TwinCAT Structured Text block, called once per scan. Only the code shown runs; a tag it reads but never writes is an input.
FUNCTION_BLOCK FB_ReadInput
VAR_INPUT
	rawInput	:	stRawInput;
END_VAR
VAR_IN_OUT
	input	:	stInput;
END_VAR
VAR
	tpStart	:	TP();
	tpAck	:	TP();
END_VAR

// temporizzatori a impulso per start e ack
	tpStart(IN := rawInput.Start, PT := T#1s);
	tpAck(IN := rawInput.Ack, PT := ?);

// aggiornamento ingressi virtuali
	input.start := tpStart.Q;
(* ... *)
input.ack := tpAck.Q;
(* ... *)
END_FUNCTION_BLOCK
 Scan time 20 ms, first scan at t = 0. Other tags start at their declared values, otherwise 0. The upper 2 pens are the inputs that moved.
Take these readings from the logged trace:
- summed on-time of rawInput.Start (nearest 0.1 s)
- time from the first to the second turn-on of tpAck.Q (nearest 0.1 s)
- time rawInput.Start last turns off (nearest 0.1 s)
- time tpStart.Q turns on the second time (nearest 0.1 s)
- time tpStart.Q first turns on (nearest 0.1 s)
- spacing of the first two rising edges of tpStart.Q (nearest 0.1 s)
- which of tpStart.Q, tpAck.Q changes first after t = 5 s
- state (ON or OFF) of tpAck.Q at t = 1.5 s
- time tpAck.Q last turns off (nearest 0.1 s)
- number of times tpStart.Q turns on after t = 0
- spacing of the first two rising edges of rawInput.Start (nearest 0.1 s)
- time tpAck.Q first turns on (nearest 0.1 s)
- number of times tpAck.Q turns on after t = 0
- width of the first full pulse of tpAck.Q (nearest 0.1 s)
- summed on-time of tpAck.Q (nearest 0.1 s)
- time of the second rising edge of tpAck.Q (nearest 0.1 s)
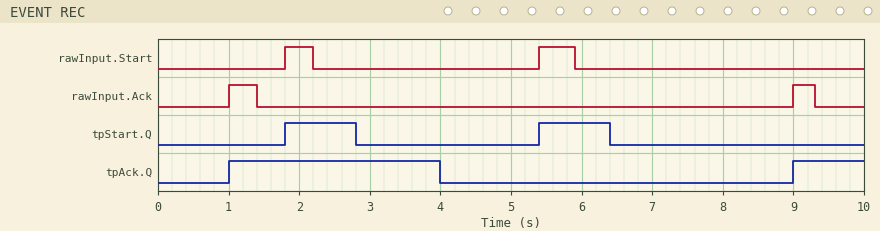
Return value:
0.9 s
8.0 s
5.9 s
5.4 s
1.8 s
3.6 s
tpStart.Q
ON
4.0 s
2
3.6 s
1.0 s
2
3.0 s
4.0 s
9.0 s
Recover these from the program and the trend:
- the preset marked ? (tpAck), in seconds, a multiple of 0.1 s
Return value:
3.0 s
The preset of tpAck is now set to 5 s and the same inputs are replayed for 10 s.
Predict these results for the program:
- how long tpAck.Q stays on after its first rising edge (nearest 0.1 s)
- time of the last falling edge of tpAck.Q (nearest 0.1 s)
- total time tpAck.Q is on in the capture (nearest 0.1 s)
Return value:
5.0 s
6.0 s
6.0 s
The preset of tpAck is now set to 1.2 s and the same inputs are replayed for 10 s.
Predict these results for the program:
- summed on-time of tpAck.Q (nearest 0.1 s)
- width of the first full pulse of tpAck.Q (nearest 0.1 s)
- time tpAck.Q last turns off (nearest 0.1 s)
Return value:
2.2 s
1.2 s
2.2 s
